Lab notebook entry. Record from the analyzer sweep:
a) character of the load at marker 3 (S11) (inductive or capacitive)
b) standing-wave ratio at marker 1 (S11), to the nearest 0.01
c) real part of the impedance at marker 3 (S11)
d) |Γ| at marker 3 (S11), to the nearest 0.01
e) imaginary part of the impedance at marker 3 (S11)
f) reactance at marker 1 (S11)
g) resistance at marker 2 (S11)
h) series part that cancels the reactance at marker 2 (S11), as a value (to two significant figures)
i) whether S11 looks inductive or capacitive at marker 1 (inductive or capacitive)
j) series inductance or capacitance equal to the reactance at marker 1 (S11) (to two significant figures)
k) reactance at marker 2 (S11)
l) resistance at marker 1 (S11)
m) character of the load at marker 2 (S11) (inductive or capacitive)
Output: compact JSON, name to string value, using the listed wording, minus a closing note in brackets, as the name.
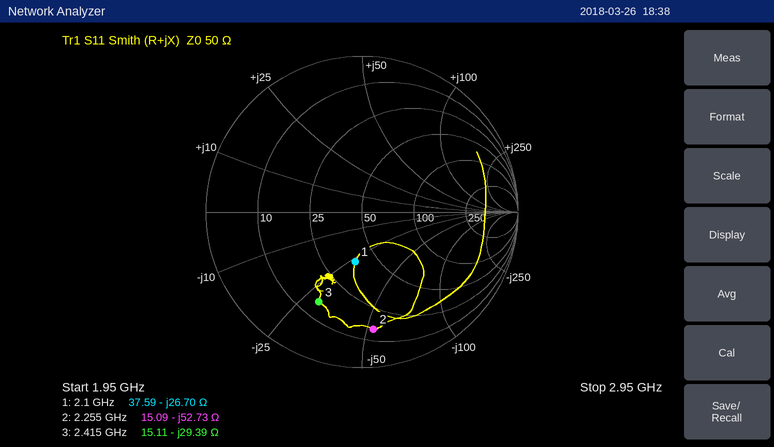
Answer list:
{"character of the load at marker 3 (S11)": "capacitive", "standing-wave ratio at marker 1 (S11), to the nearest 0.01": "1.95", "real part of the impedance at marker 3": "15.11 Ω", "|Γ| at marker 3 (S11), to the nearest 0.01": "0.64", "imaginary part of the impedance at marker 3": "-29.39 Ω", "reactance at marker 1": "-26.70 Ω", "resistance at marker 2": "15.09 Ω", "series part that cancels the reactance at marker 2 (S11), as a value": "3.7 nH", "whether S11 looks inductive or capacitive at marker 1": "capacitive", "series inductance or capacitance equal to the reactance at marker 1 (S11)": "2.8 pF", "reactance at marker 2": "-52.73 Ω", "resistance at marker 1": "37.59 Ω", "character of the load at marker 2 (S11)": "capacitive"}
